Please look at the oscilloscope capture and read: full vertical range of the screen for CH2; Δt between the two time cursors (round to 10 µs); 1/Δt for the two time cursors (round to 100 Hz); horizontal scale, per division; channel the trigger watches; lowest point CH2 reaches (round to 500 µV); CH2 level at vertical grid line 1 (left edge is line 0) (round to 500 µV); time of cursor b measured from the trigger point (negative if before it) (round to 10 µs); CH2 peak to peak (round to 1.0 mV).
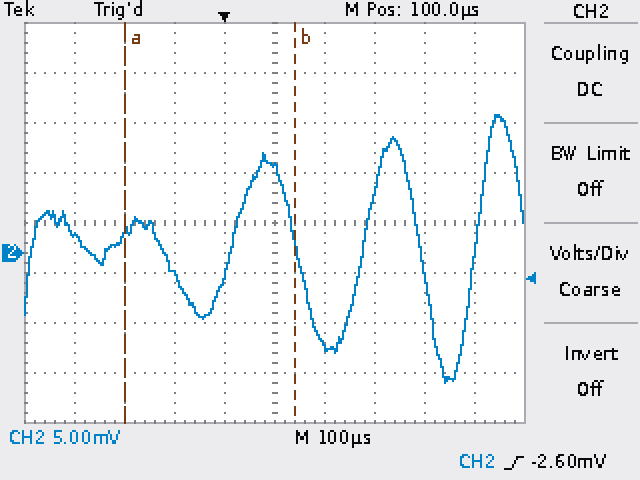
40 mV
340 µs
2.9 kHz
100 µs
CH2
-13.0 mV
2.0 mV
+140 µs
27.0 mV
